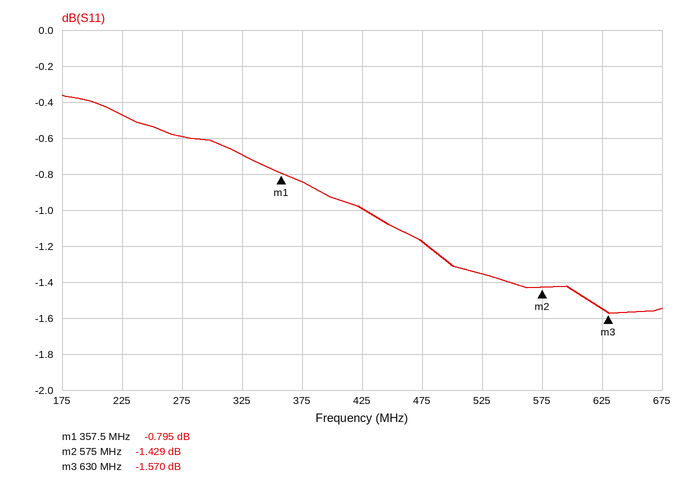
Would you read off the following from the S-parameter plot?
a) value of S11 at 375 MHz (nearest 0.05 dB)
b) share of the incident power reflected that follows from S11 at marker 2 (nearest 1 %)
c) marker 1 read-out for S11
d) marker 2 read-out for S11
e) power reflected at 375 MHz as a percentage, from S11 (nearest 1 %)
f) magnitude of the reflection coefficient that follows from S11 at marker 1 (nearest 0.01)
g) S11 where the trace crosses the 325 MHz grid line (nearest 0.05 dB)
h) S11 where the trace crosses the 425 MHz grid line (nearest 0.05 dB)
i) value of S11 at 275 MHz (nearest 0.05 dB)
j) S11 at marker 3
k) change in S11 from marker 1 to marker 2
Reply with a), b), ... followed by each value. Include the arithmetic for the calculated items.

a) -0.85 dB
b) 10^(-1.429/10) ≈ 72 %
c) -0.795 dB
d) -1.429 dB
e) 10^(-0.85/10) ≈ 82 %
f) 10^(-0.795/20) ≈ 0.91
g) -0.70 dB
h) -1.00 dB
i) -0.60 dB
j) -1.570 dB
k) -1.429 − (-0.795) = -0.634 dB
